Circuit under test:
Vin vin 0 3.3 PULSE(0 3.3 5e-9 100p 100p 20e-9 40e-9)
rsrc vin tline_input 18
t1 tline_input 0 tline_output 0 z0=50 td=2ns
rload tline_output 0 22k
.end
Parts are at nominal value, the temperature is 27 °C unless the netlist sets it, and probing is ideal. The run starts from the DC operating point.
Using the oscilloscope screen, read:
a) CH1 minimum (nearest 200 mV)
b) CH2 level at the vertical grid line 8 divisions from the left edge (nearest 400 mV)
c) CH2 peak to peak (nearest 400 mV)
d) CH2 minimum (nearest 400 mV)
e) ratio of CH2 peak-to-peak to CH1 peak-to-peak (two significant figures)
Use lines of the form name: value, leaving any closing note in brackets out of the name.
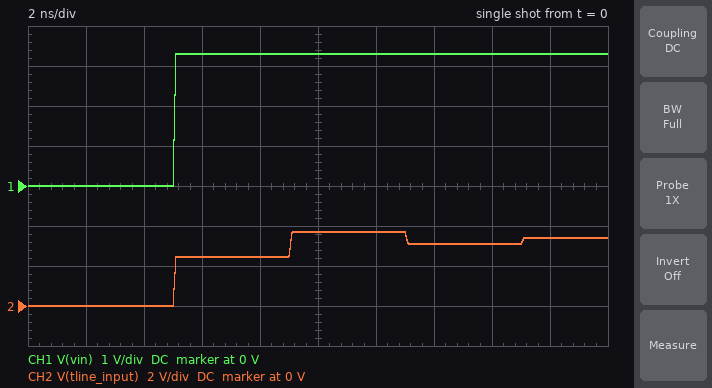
CH1 minimum: 0 V
CH2 level at the vertical grid line 8 divisions from the left edge: 3.2 V
CH2 peak to peak: 3.6 V
CH2 minimum: 0 V
ratio of CH2 peak-to-peak to CH1 peak-to-peak: 1.1
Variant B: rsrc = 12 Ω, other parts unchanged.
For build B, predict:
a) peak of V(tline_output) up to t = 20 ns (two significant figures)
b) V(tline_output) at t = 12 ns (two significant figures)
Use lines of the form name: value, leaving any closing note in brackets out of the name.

peak of V(tline_output) up to t = 20 ns: 5.3 V
V(tline_output) at t = 12 ns: 2.1 V
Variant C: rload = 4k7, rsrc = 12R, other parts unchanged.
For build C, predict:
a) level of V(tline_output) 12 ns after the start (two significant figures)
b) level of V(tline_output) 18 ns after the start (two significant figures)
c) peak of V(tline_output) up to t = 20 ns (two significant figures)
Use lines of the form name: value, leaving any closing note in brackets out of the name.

level of V(tline_output) 12 ns after the start: 2.1 V
level of V(tline_output) 18 ns after the start: 4.0 V
peak of V(tline_output) up to t = 20 ns: 5.3 V
